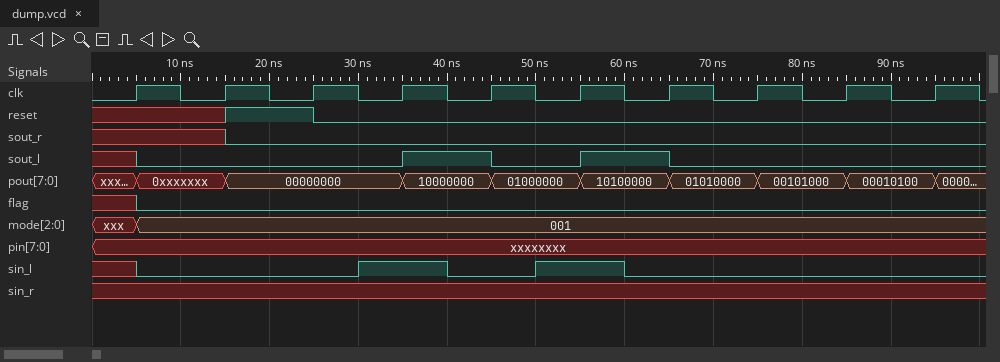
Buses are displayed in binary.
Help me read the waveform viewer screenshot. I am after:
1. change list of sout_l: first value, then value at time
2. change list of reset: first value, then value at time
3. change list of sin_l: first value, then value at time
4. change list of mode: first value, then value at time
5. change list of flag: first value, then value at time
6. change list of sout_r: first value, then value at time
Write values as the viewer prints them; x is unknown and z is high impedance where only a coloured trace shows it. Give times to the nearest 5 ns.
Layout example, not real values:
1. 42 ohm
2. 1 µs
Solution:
1. x, 0 at 5 ns, 1 at 35 ns, 0 at 45 ns, 1 at 55 ns, 0 at 65 ns
2. x, 1 at 15 ns, 0 at 25 ns
3. x, 0 at 5 ns, 1 at 30 ns, 0 at 40 ns, 1 at 50 ns, 0 at 60 ns
4. xxx, 001 at 5 ns
5. x, 0 at 5 ns
6. x, 0 at 15 ns
